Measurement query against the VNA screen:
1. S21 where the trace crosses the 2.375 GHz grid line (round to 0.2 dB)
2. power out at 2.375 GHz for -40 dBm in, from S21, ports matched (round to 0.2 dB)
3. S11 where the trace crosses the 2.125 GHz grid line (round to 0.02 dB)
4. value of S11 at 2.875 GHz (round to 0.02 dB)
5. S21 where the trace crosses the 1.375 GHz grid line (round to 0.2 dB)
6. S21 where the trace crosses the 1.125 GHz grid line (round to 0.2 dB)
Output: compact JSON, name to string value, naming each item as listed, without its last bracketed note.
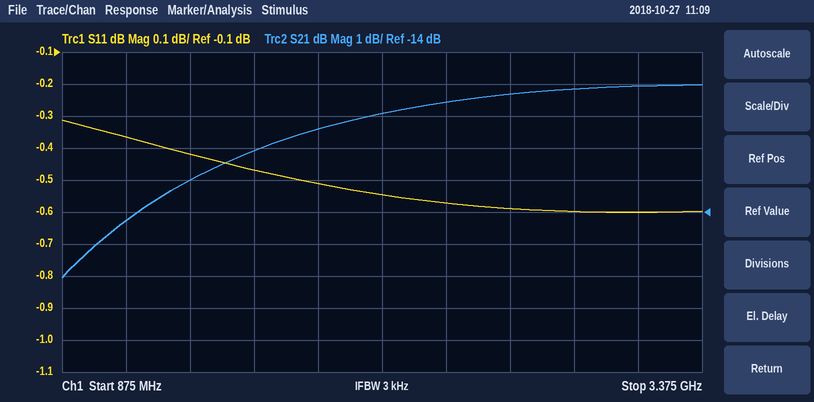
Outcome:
{"S21 where the trace crosses the 2.375 GHz grid line": "-10.6 dB", "power out at 2.375 GHz for -40 dBm in, from S21, ports matched": "-50.6 dBm", "S11 where the trace crosses the 2.125 GHz grid line": "-0.54 dB", "value of S11 at 2.875 GHz": "-0.60 dB", "S21 where the trace crosses the 1.375 GHz grid line": "-13.0 dB", "S21 where the trace crosses the 1.125 GHz grid line": "-14.2 dB"}
